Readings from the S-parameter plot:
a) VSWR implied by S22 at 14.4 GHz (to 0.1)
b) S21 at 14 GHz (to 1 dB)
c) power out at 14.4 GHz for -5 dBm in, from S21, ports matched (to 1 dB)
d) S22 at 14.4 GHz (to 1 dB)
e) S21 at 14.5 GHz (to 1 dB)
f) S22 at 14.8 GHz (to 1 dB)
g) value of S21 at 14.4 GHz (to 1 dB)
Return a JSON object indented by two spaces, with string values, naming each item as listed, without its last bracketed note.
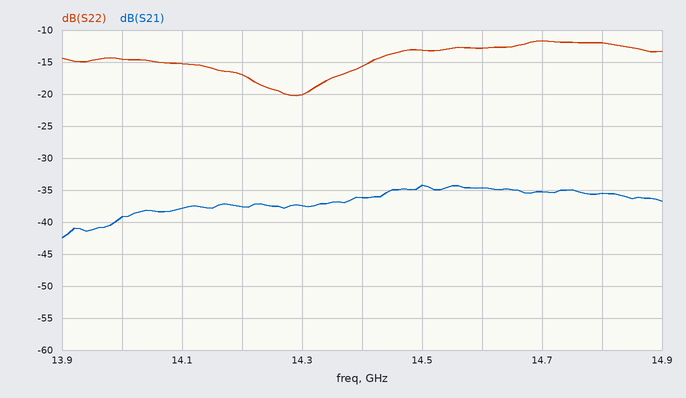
{
  "VSWR implied by S22 at 14.4 GHz": "1.4",
  "S21 at 14 GHz": "-39 dB",
  "power out at 14.4 GHz for -5 dBm in, from S21, ports matched": "-41 dBm",
  "S22 at 14.4 GHz": "-16 dB",
  "S21 at 14.5 GHz": "-34 dB",
  "S22 at 14.8 GHz": "-12 dB",
  "value of S21 at 14.4 GHz": "-36 dB"
}
